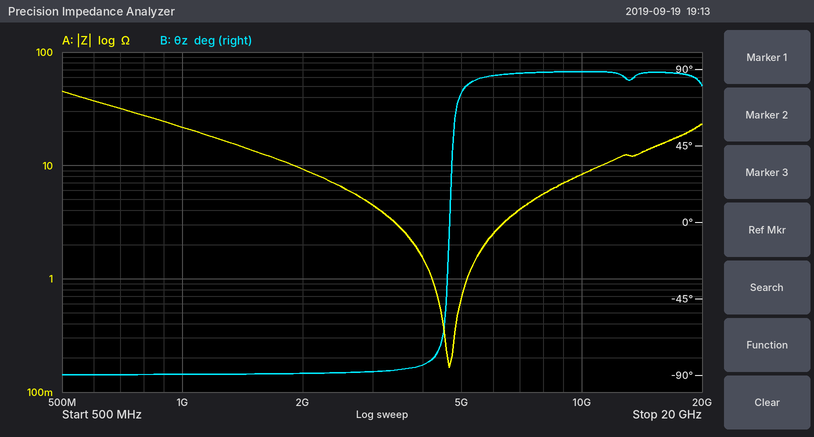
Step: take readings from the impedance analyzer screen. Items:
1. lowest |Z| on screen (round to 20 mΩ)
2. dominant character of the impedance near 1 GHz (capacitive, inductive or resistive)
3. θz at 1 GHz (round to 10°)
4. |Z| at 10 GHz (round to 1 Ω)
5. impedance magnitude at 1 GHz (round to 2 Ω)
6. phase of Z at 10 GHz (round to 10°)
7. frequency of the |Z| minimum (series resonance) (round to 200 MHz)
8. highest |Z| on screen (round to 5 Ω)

160 mΩ
capacitive
-90°
8 Ω
22 Ω
90°
4.6 GHz
45 Ω
